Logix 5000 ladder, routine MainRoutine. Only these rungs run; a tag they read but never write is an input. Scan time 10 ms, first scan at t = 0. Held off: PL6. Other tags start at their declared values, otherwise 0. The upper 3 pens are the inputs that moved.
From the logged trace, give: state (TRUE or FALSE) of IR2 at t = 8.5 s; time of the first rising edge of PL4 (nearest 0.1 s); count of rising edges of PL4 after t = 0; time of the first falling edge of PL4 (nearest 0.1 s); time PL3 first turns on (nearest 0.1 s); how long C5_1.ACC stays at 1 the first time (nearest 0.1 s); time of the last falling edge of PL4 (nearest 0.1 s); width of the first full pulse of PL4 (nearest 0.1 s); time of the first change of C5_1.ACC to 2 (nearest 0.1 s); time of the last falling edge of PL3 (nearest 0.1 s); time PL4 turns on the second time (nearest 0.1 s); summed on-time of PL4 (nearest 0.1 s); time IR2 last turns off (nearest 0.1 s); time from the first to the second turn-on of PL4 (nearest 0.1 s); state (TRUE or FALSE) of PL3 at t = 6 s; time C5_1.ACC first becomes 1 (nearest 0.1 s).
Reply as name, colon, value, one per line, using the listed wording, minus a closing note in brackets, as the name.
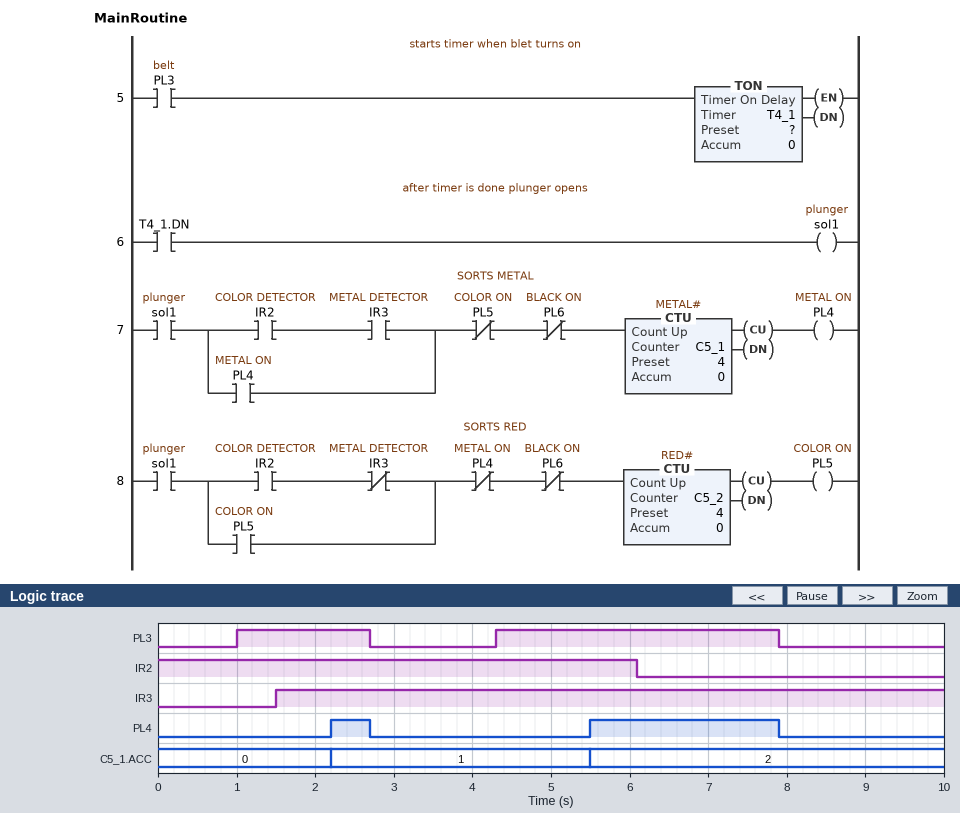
state (TRUE or FALSE) of IR2 at t = 8.5 s: FALSE
time of the first rising edge of PL4: 2.2 s
count of rising edges of PL4 after t = 0: 2
time of the first falling edge of PL4: 2.7 s
time PL3 first turns on: 1.0 s
how long C5_1.ACC stays at 1 the first time: 3.3 s
time of the last falling edge of PL4: 7.9 s
width of the first full pulse of PL4: 0.5 s
time of the first change of C5_1.ACC to 2: 5.5 s
time of the last falling edge of PL3: 7.9 s
time PL4 turns on the second time: 5.5 s
summed on-time of PL4: 2.9 s
time IR2 last turns off: 6.1 s
time from the first to the second turn-on of PL4: 3.3 s
state (TRUE or FALSE) of PL3 at t = 6 s: TRUE
time C5_1.ACC first becomes 1: 2.2 s
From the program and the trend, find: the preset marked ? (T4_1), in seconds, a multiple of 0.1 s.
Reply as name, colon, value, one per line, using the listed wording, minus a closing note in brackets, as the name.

the preset marked ? (T4_1), in seconds, a multiple of 0.1 s: 1.2 s
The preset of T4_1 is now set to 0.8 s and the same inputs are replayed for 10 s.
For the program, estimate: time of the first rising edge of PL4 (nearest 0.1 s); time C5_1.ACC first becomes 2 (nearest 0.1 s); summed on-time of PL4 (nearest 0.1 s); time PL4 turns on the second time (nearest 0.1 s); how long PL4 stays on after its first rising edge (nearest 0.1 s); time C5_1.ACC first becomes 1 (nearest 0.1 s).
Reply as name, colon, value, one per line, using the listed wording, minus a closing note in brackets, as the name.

time of the first rising edge of PL4: 1.8 s
time C5_1.ACC first becomes 2: 5.1 s
summed on-time of PL4: 3.7 s
time PL4 turns on the second time: 5.1 s
how long PL4 stays on after its first rising edge: 0.9 s
time C5_1.ACC first becomes 1: 1.8 s
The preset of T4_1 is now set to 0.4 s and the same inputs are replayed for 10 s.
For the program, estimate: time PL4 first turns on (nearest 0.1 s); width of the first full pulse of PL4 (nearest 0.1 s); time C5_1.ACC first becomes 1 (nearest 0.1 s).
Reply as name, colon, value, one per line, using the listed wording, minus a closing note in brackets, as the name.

time PL4 first turns on: 4.7 s
width of the first full pulse of PL4: 3.2 s
time C5_1.ACC first becomes 1: 4.7 s
